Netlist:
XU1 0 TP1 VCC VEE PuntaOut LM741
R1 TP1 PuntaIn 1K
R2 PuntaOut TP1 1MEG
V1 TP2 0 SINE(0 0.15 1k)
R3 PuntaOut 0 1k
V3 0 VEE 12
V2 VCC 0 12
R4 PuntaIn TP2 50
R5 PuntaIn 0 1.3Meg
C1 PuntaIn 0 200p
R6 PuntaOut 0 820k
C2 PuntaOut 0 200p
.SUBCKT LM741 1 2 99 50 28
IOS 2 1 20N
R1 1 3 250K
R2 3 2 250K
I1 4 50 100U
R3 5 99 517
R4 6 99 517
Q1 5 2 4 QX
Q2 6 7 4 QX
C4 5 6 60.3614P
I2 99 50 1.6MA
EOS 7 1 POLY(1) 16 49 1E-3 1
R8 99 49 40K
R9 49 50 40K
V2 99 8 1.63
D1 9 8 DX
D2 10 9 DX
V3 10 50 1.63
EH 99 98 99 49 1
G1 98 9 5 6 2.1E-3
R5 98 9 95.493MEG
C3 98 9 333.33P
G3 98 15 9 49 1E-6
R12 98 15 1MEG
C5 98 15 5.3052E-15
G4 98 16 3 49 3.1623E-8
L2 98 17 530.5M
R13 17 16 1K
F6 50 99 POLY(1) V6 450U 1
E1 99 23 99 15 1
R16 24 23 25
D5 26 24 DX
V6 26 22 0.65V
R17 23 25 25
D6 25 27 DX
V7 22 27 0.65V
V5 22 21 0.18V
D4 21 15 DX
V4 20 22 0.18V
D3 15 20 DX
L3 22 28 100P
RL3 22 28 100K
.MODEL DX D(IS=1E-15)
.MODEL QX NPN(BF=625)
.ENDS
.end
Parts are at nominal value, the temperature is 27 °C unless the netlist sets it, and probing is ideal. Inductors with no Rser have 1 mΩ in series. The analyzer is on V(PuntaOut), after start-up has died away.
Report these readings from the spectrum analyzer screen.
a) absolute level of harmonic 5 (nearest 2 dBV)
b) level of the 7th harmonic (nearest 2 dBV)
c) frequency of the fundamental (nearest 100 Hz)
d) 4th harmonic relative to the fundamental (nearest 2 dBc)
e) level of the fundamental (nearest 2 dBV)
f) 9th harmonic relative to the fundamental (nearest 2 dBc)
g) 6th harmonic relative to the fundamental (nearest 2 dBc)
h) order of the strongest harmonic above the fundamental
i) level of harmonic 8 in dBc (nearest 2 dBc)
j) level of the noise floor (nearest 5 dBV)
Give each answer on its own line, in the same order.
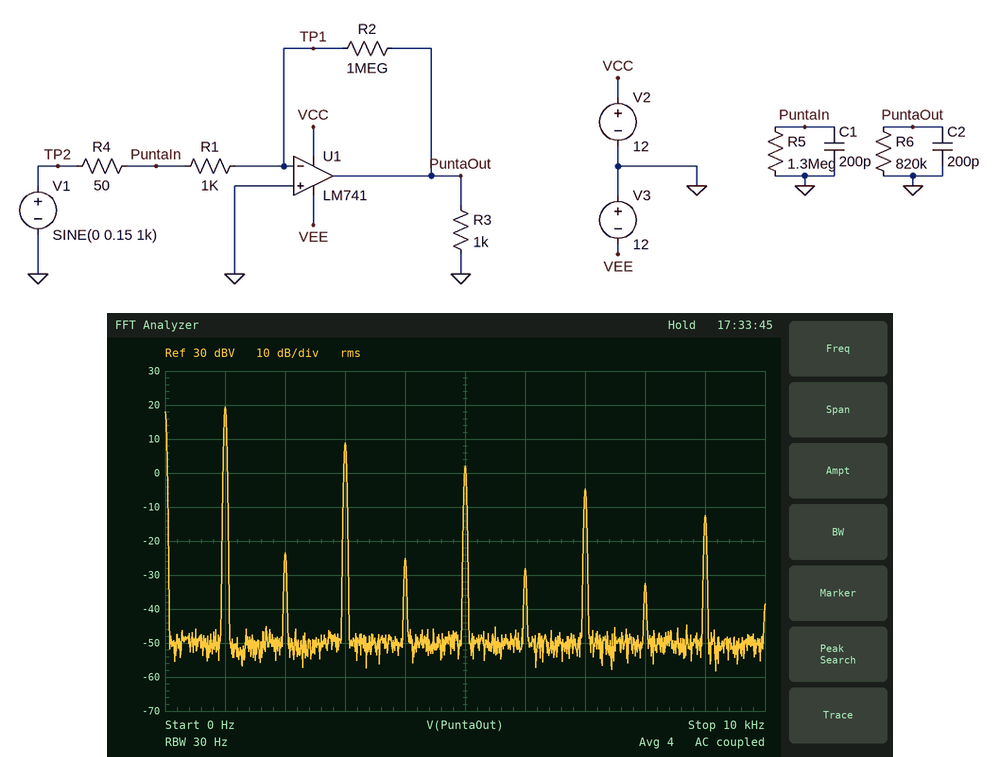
2 dBV
-4 dBV
1.0 kHz
-44 dBc
20 dBV
-32 dBc
-48 dBc
3
-52 dBc
-50 dBV
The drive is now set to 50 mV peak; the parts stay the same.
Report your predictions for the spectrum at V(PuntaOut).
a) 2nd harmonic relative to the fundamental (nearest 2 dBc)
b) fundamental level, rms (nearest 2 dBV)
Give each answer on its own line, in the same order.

-34 dBc
20 dBV
